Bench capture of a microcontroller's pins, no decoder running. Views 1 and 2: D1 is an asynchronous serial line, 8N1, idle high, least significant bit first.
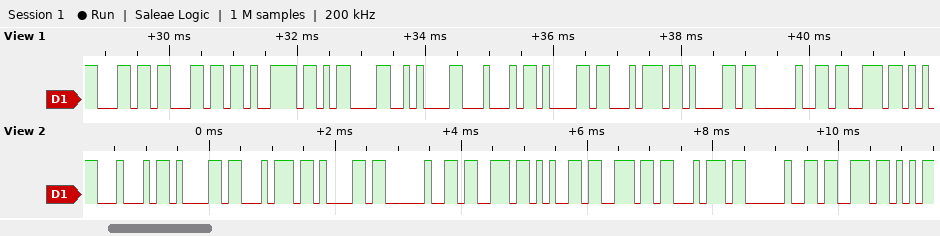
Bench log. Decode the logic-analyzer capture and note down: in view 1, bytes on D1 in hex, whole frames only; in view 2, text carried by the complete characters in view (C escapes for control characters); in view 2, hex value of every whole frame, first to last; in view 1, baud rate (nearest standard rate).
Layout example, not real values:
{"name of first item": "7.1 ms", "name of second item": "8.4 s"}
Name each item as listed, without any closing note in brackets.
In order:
{"in view 1, bytes on D1 in hex, whole frames only": "6C 6C 79 0D 0A 44 61 74 61 20 73", "in view 2, text carried by the complete characters in view": "\"Data sent s\"", "in view 2, hex value of every whole frame, first to last": "44 61 74 61 20 73 65 6E 74 20 73", "in view 1, baud rate": "9600 baud"}
